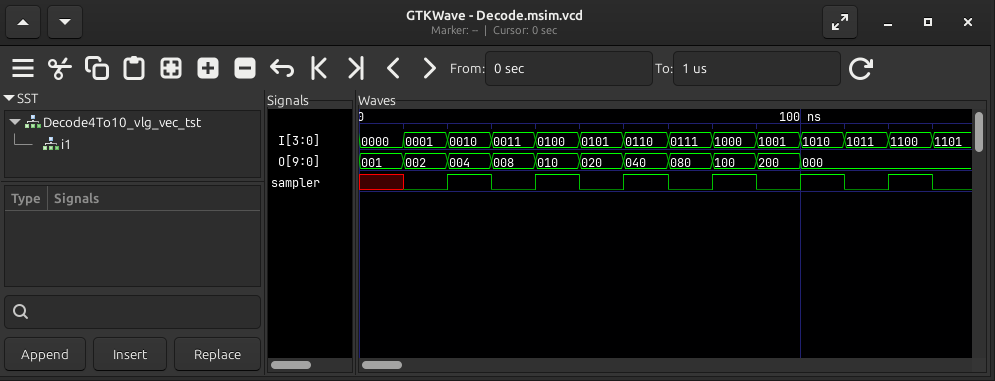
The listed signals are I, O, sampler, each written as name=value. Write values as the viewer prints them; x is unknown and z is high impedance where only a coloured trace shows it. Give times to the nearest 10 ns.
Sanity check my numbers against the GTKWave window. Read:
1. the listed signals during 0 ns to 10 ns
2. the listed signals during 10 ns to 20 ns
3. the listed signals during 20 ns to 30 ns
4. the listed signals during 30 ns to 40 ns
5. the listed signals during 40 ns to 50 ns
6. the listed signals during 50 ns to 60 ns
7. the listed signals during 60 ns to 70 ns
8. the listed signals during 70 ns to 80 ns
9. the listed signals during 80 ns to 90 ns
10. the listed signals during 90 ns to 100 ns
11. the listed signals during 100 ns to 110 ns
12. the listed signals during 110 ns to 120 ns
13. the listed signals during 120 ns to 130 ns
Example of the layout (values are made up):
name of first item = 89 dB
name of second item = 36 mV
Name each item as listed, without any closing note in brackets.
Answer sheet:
the listed signals during 0 ns to 10 ns = I=0000, O=001, sampler=x
the listed signals during 10 ns to 20 ns = I=0001, O=002, sampler=0
the listed signals during 20 ns to 30 ns = I=0010, O=004, sampler=1
the listed signals during 30 ns to 40 ns = I=0011, O=008, sampler=0
the listed signals during 40 ns to 50 ns = I=0100, O=010, sampler=1
the listed signals during 50 ns to 60 ns = I=0101, O=020, sampler=0
the listed signals during 60 ns to 70 ns = I=0110, O=040, sampler=1
the listed signals during 70 ns to 80 ns = I=0111, O=080, sampler=0
the listed signals during 80 ns to 90 ns = I=1000, O=100, sampler=1
the listed signals during 90 ns to 100 ns = I=1001, O=200, sampler=0
the listed signals during 100 ns to 110 ns = I=1010, O=000, sampler=1
the listed signals during 110 ns to 120 ns = I=1011, O=000, sampler=0
the listed signals during 120 ns to 130 ns = I=1100, O=000, sampler=1
